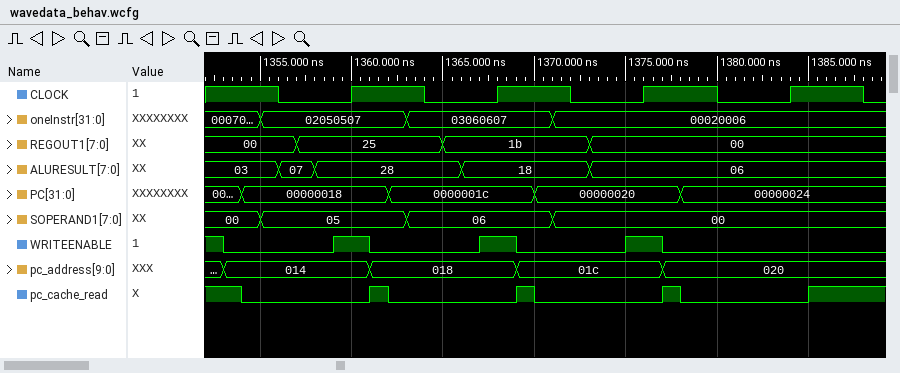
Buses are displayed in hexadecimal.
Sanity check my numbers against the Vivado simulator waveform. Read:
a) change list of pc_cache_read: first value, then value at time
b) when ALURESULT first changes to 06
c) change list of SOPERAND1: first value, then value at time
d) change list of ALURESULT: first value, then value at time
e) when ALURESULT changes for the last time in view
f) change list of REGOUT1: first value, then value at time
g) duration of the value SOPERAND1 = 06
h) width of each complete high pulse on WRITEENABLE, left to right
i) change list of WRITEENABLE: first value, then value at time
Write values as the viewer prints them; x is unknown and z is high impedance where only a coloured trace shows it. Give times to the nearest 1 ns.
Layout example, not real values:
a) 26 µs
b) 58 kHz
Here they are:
a) 1, 0 at 1354 ns, 1 at 1361 ns, 0 at 1362 ns, 1 at 1369 ns, 0 at 1370 ns, 1 at 1377 ns, 0 at 1378 ns, 1 at 1385 ns
b) 1373 ns
c) 00, 05 at 1355 ns, 06 at 1363 ns, 00 at 1371 ns
d) 03, 07 at 1356 ns, 28 at 1358 ns, 18 at 1366 ns, 06 at 1373 ns
e) 1373 ns
f) 00, 25 at 1357 ns, 1b at 1365 ns, 00 at 1373 ns
g) 8 ns
h) 2 ns, 2 ns, 2 ns
i) 1, 0 at 1353 ns, 1 at 1359 ns, 0 at 1361 ns, 1 at 1367 ns, 0 at 1369 ns, 1 at 1375 ns, 0 at 1377 ns
